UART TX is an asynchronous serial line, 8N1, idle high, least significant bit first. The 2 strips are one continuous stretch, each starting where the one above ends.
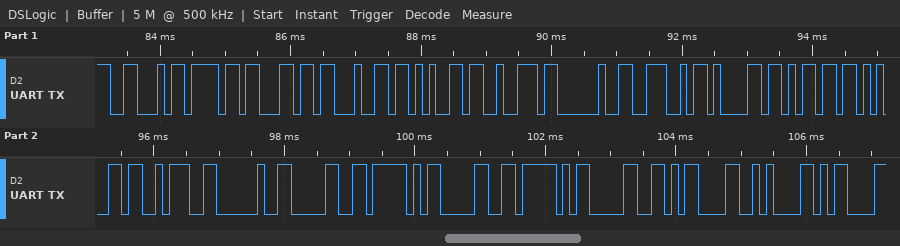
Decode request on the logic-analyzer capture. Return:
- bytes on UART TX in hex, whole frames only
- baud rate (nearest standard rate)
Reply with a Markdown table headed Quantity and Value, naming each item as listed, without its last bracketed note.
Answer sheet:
| Quantity | Value |
|---|---|
| bytes on UART TX in hex, whole frames only | 0x46 0x6F 0x6C 0x64 0x65 0x72 0x20 0x4E 0x61 0x6D 0x65 0x3A 0x20 0x30 0x5F 0x30 0x5F 0x30 0x0D 0x0A 0x0D |
| baud rate | 9600 baud |
